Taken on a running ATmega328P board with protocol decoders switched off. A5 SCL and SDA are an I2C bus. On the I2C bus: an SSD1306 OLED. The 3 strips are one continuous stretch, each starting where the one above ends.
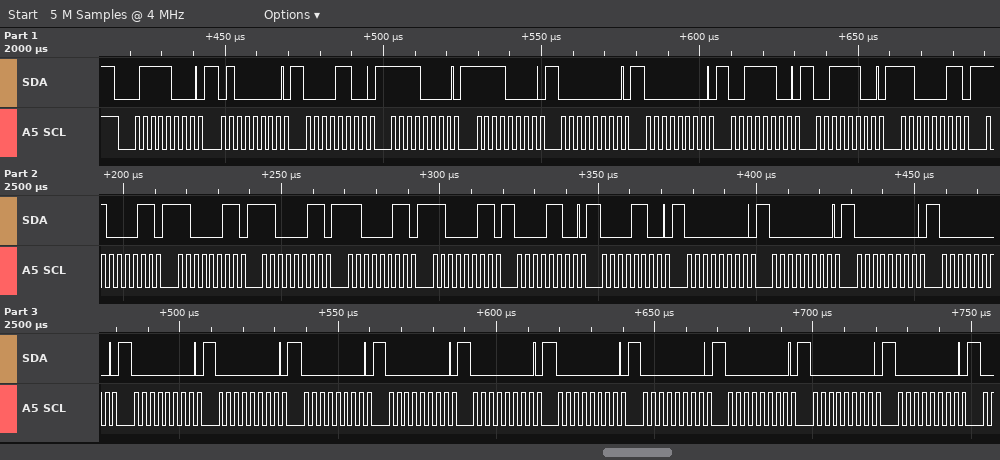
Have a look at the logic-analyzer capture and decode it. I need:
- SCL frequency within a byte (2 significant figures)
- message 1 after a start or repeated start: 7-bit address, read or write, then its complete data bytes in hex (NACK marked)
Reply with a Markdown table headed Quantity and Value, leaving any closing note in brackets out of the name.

| Quantity | Value |
|---|---|
| SCL frequency within a byte | 400 kHz |
| message 1 after a start or repeated start: 7-bit address, read or write, then its complete data bytes in hex | 0x3C write: 40 0C F0 F0 00 00 3C 3C C3 C3 C3 C3 C3 C3 0C 0C 00 00 00 00 00 00 00 00 00 00 00 00 00 00 |
